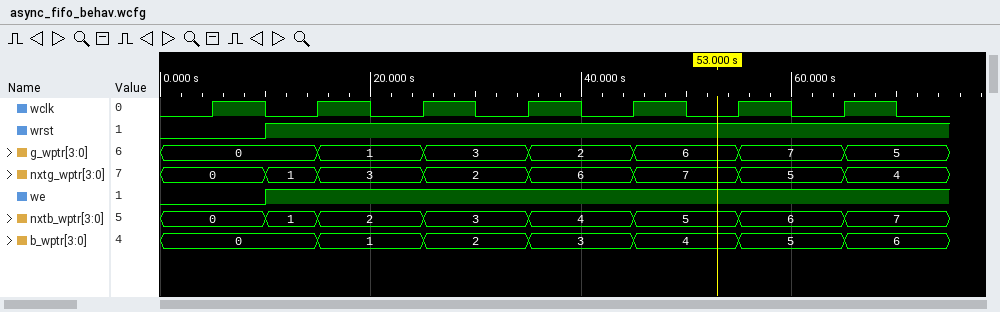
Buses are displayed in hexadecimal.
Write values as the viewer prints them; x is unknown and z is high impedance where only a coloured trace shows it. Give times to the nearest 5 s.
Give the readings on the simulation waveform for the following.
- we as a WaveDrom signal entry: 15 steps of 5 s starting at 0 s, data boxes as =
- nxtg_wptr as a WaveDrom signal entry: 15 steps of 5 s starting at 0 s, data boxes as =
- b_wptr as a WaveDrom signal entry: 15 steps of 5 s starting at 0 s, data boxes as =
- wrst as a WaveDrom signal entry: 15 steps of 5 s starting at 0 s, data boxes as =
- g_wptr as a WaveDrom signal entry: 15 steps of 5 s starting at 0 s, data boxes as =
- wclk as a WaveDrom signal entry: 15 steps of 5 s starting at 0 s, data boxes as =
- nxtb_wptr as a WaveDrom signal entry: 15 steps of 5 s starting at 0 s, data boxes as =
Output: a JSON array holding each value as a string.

["{name: 'we', wave: '0.1............'}", "{name: 'nxtg_wptr', wave: '=.==.=.=.=.=.=.', data: '0 1 3 2 6 7 5 4'}", "{name: 'b_wptr', wave: '=..=.=.=.=.=.=.', data: '0 1 2 3 4 5 6'}", "{name: 'wrst', wave: '0.1............'}", "{name: 'g_wptr', wave: '=..=.=.=.=.=.=.', data: '0 1 3 2 6 7 5'}", "{name: 'wclk', wave: '010101010101010'}", "{name: 'nxtb_wptr', wave: '=.==.=.=.=.=.=.', data: '0 1 2 3 4 5 6 7'}"]
